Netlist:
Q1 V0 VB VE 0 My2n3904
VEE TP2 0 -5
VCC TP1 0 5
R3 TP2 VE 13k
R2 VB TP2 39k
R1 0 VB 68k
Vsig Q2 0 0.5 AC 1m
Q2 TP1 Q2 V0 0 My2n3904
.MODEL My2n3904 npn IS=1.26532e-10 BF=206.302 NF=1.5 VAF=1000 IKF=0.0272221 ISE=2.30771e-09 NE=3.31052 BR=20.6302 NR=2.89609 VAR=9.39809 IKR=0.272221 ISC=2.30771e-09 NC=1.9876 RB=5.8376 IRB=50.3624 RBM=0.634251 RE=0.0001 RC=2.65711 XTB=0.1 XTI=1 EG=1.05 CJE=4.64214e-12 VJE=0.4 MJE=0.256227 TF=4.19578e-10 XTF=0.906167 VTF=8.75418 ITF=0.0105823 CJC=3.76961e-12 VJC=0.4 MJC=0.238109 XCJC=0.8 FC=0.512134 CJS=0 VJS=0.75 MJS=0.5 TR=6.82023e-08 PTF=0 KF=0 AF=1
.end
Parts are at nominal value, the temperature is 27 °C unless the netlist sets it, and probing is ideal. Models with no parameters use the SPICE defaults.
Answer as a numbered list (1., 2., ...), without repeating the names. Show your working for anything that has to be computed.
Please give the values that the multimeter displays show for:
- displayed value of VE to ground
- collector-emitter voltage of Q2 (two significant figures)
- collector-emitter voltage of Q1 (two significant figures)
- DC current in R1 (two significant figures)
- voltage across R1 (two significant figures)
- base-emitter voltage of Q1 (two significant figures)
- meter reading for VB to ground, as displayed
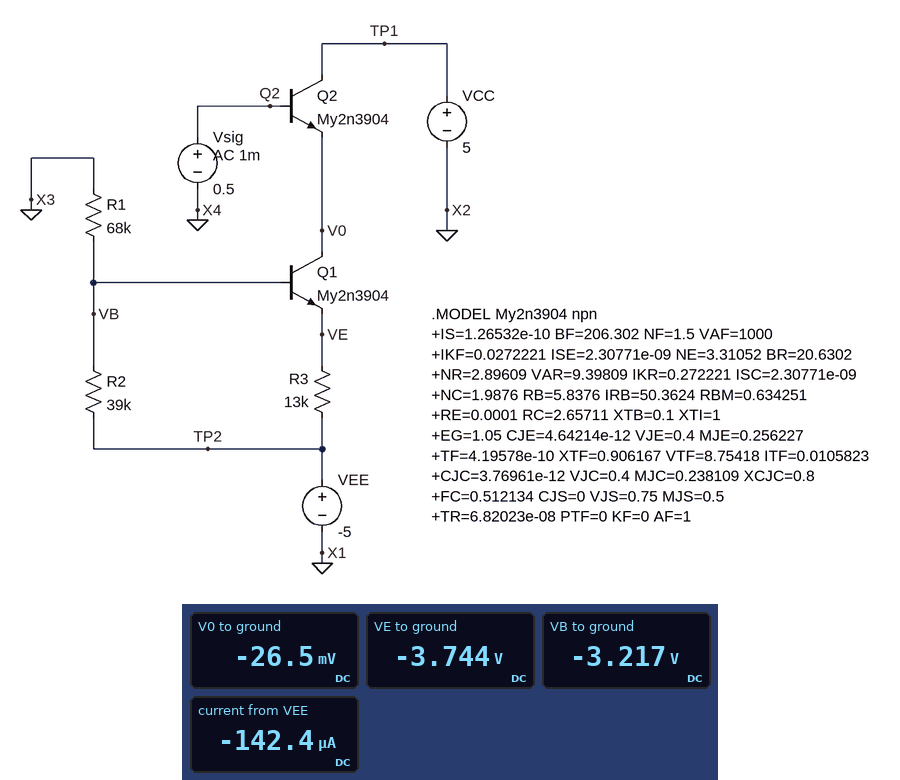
1. -3.744 V
2. 5 V - (-26.5 mV) = 5.0 V
3. -26.5 mV - (-3.744 V) = 3.7 V
4. (0 V - (-3.217 V)) / 68 kΩ = 47 µA
5. 0 V - (-3.217 V) = 3.2 V
6. -3.217 V - (-3.744 V) = 530 mV
7. -3.217 V
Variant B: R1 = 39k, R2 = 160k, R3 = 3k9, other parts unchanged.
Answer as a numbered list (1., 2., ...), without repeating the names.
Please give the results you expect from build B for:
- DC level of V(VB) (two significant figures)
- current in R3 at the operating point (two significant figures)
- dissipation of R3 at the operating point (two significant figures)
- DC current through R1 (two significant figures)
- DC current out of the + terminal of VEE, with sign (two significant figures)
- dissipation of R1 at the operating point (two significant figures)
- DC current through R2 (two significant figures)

1. -1.2 V
2. 820 µA
3. 2.6 mW
4. 31 µA
5. -840 µA
6. 37 µW
7. 24 µA
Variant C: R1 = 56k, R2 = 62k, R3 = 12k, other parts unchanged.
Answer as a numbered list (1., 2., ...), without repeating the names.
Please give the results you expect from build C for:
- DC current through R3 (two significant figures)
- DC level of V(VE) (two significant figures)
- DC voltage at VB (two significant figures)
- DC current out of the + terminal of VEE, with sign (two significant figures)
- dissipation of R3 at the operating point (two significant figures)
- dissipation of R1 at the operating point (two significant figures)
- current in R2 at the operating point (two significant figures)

1. 170 µA
2. -3.0 V
3. -2.4 V
4. -210 µA
5. 340 µW
6. 110 µW
7. 41 µA
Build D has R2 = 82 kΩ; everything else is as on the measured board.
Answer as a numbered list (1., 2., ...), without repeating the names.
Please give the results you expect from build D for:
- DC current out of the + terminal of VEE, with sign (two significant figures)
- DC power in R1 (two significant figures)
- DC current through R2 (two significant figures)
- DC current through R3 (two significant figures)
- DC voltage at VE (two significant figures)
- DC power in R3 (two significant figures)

1. -190 µA
2. 81 µW
3. 32 µA
4. 160 µA
5. -2.9 V
6. 340 µW
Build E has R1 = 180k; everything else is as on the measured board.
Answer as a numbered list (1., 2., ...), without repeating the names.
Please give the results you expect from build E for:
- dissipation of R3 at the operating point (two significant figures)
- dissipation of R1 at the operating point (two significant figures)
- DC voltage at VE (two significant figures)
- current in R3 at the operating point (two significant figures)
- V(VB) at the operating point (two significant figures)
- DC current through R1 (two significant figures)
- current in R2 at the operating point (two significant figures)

1. 11 µW
2. 95 µW
3. -4.6 V
4. 30 µA
5. -4.1 V
6. 23 µA
7. 22 µA
